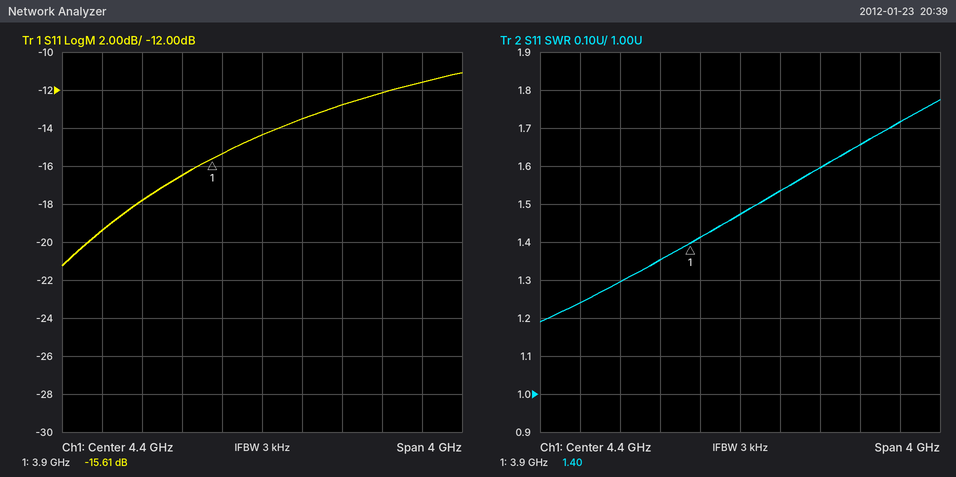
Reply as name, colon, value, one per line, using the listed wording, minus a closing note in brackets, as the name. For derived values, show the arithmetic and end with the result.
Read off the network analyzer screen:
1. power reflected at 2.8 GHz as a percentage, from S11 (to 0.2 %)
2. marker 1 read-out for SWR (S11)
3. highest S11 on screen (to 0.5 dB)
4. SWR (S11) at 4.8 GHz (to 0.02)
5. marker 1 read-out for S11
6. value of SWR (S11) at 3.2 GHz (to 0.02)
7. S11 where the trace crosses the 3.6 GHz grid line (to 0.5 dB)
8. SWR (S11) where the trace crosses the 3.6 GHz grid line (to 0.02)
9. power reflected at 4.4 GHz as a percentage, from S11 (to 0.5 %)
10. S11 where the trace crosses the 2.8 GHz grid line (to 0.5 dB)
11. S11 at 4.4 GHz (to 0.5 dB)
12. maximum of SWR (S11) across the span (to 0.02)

power reflected at 2.8 GHz as a percentage, from S11: 10^(-19.5/10) ≈ 1.12 %, so 1.2 % to the nearest 0.2 %
marker 1 read-out for SWR: 1.40
highest S11 on screen: -11.0 dB
SWR (S11) at 4.8 GHz: 1.54
marker 1 read-out for S11: -15.61 dB
value of SWR (S11) at 3.2 GHz: 1.30
S11 where the trace crosses the 3.6 GHz grid line: -16.5 dB
SWR (S11) where the trace crosses the 3.6 GHz grid line: 1.36
power reflected at 4.4 GHz as a percentage, from S11: 10^(-14.5/10) ≈ 3.5 %
S11 where the trace crosses the 2.8 GHz grid line: -19.5 dB
S11 at 4.4 GHz: -14.5 dB
maximum of SWR (S11) across the span: 1.78
